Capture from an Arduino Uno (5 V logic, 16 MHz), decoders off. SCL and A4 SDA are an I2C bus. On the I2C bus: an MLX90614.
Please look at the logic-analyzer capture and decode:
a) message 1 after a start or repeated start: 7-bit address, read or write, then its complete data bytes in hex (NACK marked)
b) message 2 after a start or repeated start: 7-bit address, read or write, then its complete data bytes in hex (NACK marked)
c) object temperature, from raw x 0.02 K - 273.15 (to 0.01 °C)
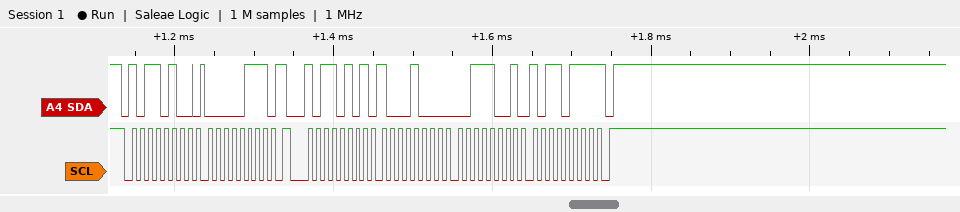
0x5A write: 07
0x5A read: 88 39 B7 NACK
21.41 °C
